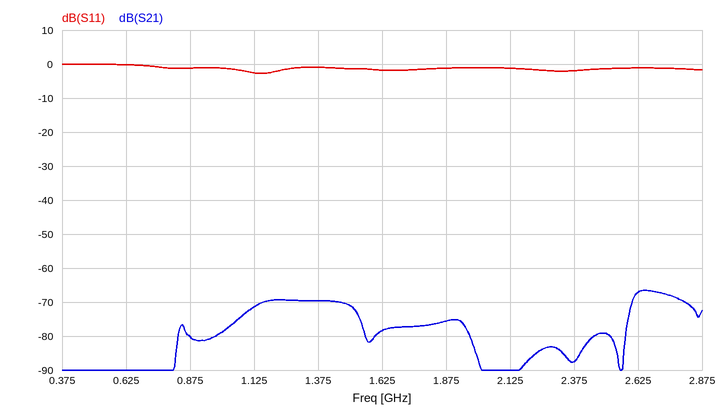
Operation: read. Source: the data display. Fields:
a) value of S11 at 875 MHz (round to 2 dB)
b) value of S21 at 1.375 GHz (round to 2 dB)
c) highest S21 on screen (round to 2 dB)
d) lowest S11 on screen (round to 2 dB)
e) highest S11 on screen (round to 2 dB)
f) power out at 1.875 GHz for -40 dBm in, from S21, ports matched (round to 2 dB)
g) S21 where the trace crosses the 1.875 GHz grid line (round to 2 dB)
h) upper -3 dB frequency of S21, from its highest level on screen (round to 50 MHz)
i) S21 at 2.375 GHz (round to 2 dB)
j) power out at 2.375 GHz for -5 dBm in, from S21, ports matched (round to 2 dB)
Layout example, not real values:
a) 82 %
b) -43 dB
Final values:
a) -2 dB
b) -70 dB
c) -66 dB
d) -2 dB
e) 0 dB
f) -116 dBm
g) -76 dB
h) 2.80 GHz
i) -88 dB
j) -92 dBm
